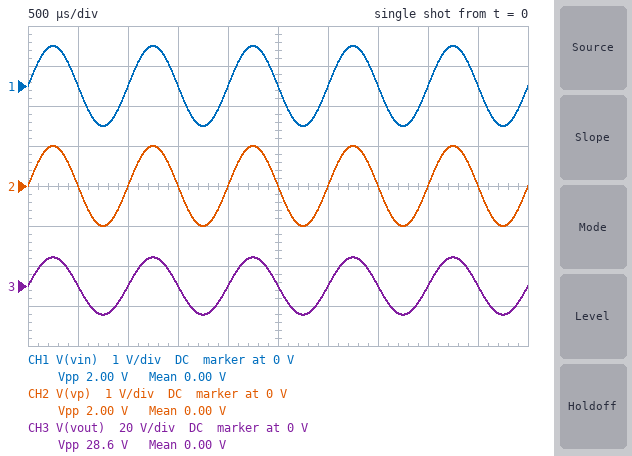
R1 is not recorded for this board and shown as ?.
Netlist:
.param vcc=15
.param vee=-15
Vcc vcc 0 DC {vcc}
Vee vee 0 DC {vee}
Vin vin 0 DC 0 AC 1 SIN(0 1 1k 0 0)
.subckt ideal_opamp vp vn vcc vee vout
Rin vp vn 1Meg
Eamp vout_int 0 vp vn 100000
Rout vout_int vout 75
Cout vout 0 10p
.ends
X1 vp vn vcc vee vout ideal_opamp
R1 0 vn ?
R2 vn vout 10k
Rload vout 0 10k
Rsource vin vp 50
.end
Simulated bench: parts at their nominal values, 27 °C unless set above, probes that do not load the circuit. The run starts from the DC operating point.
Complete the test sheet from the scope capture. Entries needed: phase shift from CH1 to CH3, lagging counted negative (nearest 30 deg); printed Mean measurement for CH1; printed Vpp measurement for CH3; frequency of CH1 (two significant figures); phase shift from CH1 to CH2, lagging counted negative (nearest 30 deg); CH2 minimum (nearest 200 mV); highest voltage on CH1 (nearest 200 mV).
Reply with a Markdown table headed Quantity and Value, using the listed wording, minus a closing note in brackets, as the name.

| Quantity | Value |
|---|---|
| phase shift from CH1 to CH3, lagging counted negative | 0 deg |
| printed Mean measurement for CH1 | 0.00 V |
| printed Vpp measurement for CH3 | 28.6 V |
| frequency of CH1 | 1.0 kHz |
| phase shift from CH1 to CH2, lagging counted negative | 0 deg |
| CH2 minimum | -1.0 V |
| highest voltage on CH1 | 1.0 V |
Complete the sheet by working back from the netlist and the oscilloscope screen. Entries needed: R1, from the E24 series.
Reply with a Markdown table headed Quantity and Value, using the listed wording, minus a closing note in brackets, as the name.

| Quantity | Value |
|---|---|
| R1, from the E24 series | 750 Ω |
